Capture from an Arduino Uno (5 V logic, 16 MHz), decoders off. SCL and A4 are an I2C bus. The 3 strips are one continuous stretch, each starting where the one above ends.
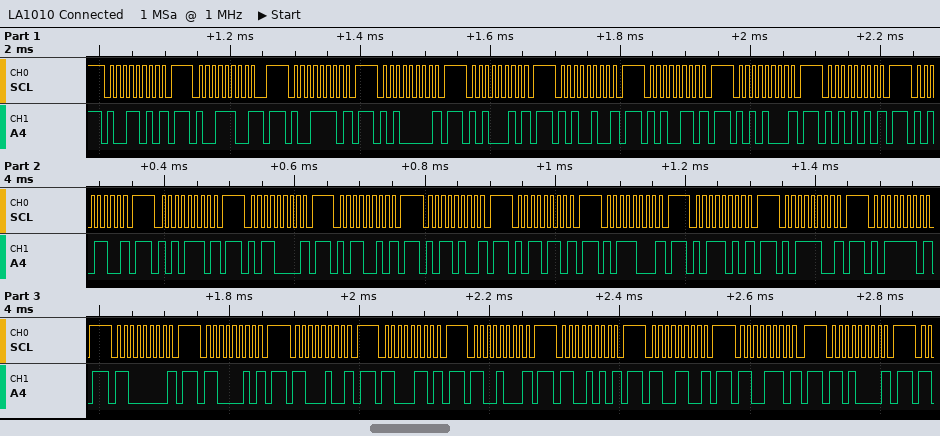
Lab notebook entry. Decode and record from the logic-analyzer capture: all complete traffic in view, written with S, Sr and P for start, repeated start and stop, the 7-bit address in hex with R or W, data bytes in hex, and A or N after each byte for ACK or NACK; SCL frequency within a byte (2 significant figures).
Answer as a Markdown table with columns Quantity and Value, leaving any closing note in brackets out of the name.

| Quantity | Value |
|---|---|
| all complete traffic in view, written with S, Sr and P for start, repeated start and stop, the 7-bit address in hex with R or W, data bytes in hex, and A or N after each byte for ACK or NACK | S 4DW N P S 4EW N P S 4FW N P S 50W N P S 51W N P S 52W N P S 53W N P S 54W N P S 55W N P S 56W N P S 57W N P S 58W N P S 59W N P S 5AW N P S 5BW N P S 5CW N P S 5DW N P S 5EW N P S 5FW N P S 60W N P S 61W N P S 62W N P S 63W N P S 64W N P S 65W N P S 66W N P S 67W N P S 68W N P |
| SCL frequency within a byte | 100 kHz |
